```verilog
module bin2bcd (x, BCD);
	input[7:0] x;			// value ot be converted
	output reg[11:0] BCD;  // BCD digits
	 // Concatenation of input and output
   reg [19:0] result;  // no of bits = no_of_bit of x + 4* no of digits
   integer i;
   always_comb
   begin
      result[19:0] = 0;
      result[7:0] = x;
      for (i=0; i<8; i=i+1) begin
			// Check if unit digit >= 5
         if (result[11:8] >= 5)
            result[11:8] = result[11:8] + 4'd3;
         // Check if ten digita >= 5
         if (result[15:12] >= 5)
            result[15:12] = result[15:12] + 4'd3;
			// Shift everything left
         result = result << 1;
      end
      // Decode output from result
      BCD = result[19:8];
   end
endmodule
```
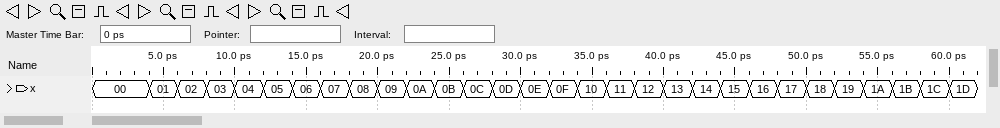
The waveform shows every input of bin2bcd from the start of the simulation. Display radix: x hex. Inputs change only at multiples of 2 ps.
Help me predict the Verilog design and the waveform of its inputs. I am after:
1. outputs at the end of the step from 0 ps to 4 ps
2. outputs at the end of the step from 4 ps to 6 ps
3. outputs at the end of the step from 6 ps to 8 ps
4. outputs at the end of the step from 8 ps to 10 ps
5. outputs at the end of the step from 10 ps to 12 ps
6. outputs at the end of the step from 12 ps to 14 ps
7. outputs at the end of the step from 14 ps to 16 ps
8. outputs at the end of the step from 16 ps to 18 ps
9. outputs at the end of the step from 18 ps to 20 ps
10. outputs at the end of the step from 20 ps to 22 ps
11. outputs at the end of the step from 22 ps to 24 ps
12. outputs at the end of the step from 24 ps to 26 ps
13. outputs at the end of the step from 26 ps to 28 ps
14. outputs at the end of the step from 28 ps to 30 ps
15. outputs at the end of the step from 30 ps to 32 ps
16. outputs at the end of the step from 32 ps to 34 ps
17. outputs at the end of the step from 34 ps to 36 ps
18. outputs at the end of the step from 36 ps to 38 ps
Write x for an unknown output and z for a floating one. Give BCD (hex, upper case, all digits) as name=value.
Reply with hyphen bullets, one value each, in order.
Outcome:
- BCD=000
- BCD=001
- BCD=002
- BCD=003
- BCD=004
- BCD=005
- BCD=006
- BCD=007
- BCD=008
- BCD=009
- BCD=010
- BCD=011
- BCD=012
- BCD=013
- BCD=014
- BCD=015
- BCD=016
- BCD=017
